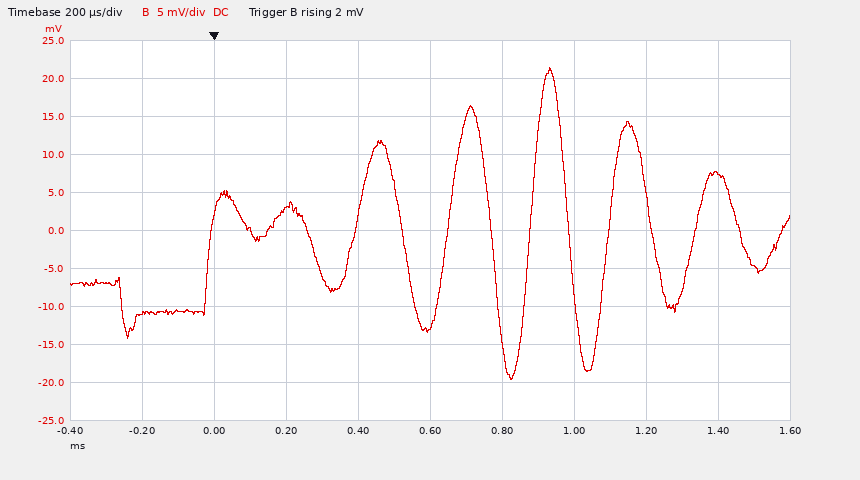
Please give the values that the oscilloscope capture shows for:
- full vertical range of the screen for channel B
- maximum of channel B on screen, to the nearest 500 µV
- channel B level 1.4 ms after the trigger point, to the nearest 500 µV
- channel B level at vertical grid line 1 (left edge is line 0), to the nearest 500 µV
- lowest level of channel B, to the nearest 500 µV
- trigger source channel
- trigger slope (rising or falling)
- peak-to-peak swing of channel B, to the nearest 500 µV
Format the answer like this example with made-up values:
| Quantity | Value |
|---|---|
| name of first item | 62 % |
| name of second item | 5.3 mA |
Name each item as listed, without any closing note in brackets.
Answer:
| Quantity | Value |
|---|---|
| full vertical range of the screen for channel B | 50 mV |
| maximum of channel B on screen, to the nearest 500 µV | 21.5 mV |
| channel B level 1.4 ms after the trigger point, to the nearest 500 µV | 7.5 mV |
| channel B level at vertical grid line 1 (left edge is line 0), to the nearest 500 µV | -11.0 mV |
| lowest level of channel B, to the nearest 500 µV | -19.5 mV |
| trigger source channel | channel B |
| trigger slope | rising |
| peak-to-peak swing of channel B, to the nearest 500 µV | 41.0 mV |
